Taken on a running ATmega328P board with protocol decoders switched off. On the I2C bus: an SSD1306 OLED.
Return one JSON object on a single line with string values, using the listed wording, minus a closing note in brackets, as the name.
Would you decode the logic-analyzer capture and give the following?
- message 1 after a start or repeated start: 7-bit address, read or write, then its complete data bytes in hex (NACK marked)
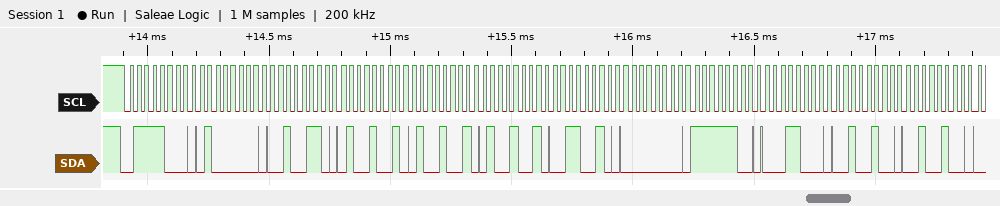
{"message 1 after a start or repeated start: 7-bit address, read or write, then its complete data bytes in hex": "0x3C write: 40 26 49 49 49 32 00 FC 18 24 24"}
